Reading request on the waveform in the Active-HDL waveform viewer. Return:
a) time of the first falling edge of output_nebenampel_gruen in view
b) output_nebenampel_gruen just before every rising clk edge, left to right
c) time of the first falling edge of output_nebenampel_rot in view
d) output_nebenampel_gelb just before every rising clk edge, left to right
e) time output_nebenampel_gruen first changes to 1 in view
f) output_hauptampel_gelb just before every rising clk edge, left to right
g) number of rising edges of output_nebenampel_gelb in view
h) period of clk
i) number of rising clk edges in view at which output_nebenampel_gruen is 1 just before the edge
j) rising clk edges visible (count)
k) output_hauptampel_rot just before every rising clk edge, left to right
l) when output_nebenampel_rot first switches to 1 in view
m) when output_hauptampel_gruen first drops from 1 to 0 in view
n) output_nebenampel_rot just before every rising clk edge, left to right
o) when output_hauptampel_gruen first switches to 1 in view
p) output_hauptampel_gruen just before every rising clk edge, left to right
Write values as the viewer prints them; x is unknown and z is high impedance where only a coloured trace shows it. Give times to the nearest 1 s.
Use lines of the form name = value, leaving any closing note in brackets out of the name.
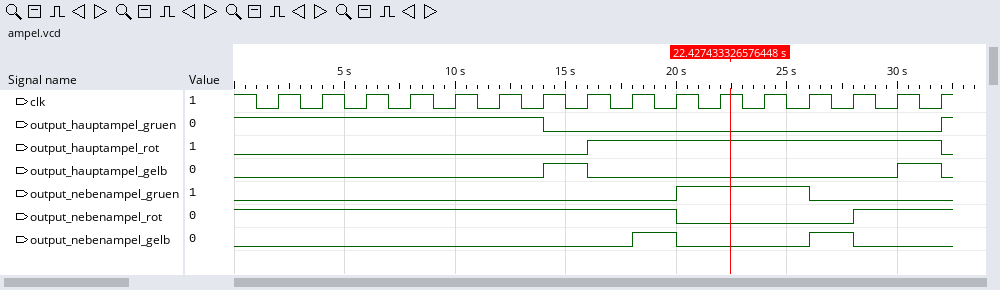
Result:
time of the first falling edge of output_nebenampel_gruen in view = 26 s
output_nebenampel_gruen just before every rising clk edge, left to right = 0 0 0 0 0 0 0 0 0 0 1 1 1 0 0 0
time of the first falling edge of output_nebenampel_rot in view = 20 s
output_nebenampel_gelb just before every rising clk edge, left to right = 0 0 0 0 0 0 0 0 0 1 0 0 0 1 0 0
time output_nebenampel_gruen first changes to 1 in view = 20 s
output_hauptampel_gelb just before every rising clk edge, left to right = 0 0 0 0 0 0 0 1 0 0 0 0 0 0 0 1
number of rising edges of output_nebenampel_gelb in view = 2
period of clk = 2 s
number of rising clk edges in view at which output_nebenampel_gruen is 1 just before the edge = 3
rising clk edges visible = 16
output_hauptampel_rot just before every rising clk edge, left to right = 0 0 0 0 0 0 0 0 1 1 1 1 1 1 1 1
when output_nebenampel_rot first switches to 1 in view = 28 s
when output_hauptampel_gruen first drops from 1 to 0 in view = 14 s
output_nebenampel_rot just before every rising clk edge, left to right = 1 1 1 1 1 1 1 1 1 1 0 0 0 0 1 1
when output_hauptampel_gruen first switches to 1 in view = 32 s
output_hauptampel_gruen just before every rising clk edge, left to right = 1 1 1 1 1 1 1 0 0 0 0 0 0 0 0 0
